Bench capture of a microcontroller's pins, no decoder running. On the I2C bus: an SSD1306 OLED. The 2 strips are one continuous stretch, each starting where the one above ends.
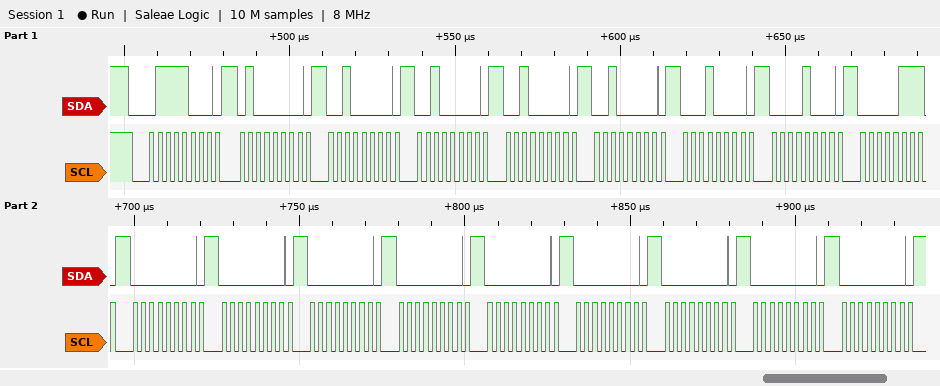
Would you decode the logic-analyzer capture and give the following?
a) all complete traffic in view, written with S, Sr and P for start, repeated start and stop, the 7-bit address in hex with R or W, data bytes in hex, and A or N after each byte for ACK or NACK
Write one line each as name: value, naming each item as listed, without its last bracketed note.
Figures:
all complete traffic in view, written with S, Sr and P for start, repeated start and stop, the 7-bit address in hex with R or W, data bytes in hex, and A or N after each byte for ACK or NACK: S 3CW A 40 A 20 A 20 A 20 A 20 A 10 A 08 A 07 A 00 A 00 A 00 A 00 A 00 A 00 A 00 A 00 A 00 A
